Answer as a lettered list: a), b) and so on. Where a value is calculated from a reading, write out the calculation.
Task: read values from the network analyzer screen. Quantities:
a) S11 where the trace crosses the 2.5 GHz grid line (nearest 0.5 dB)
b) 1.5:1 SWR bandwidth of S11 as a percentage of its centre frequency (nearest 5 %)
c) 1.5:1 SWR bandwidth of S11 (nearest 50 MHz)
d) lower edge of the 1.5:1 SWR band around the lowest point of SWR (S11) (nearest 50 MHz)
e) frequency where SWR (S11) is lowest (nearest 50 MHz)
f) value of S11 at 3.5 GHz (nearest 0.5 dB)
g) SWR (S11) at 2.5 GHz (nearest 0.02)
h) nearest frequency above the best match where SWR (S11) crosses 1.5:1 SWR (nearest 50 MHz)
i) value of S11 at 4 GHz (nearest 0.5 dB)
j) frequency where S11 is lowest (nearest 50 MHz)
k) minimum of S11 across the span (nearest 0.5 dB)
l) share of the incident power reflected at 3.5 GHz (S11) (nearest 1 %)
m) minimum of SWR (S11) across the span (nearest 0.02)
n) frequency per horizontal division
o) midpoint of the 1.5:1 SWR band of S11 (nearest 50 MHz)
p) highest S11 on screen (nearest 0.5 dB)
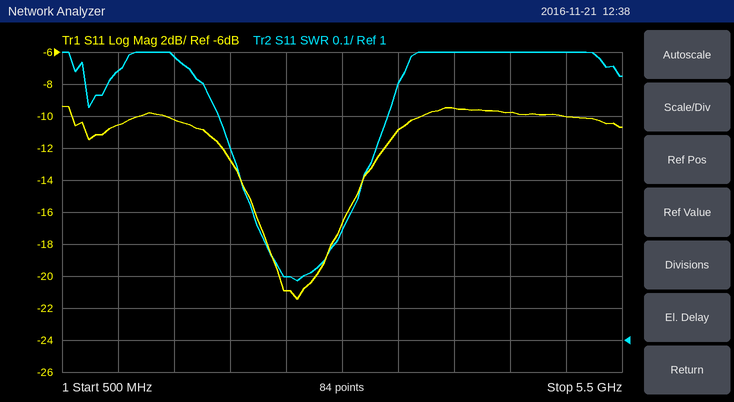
a) -21.0 dB
b) 1.1 GHz / 2.65 GHz ≈ 41.5 %, so 40 % to the nearest 5 %
c) 3.20 GHz − 2.10 GHz = 1.10 GHz
d) 2.10 GHz
e) 2.60 GHz
f) -11.0 dB
g) 1.20
h) 3.20 GHz
i) -9.5 dB
j) 2.60 GHz
k) -21.5 dB
l) 10^(-11/10) ≈ 8 %
m) 1.18
n) 500 MHz
o) 2.65 GHz
p) -9.5 dB
